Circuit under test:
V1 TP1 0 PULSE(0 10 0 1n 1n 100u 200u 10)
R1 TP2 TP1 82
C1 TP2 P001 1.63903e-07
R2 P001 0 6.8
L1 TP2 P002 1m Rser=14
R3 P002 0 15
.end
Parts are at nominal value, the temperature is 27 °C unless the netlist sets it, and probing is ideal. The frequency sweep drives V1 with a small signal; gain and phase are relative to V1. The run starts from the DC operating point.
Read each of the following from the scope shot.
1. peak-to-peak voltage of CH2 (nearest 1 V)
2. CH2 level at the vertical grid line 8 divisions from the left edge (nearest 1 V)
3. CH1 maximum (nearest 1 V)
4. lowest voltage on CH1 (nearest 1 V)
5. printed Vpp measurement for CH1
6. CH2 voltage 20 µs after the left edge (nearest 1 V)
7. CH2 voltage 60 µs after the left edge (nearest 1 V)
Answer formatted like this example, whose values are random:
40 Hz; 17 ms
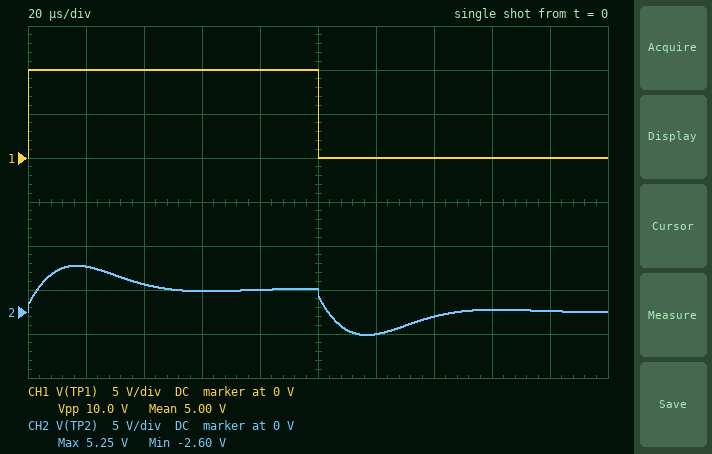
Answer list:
8 V; 0 V; 10 V; 0 V; 10.0 V; 5 V; 2 V
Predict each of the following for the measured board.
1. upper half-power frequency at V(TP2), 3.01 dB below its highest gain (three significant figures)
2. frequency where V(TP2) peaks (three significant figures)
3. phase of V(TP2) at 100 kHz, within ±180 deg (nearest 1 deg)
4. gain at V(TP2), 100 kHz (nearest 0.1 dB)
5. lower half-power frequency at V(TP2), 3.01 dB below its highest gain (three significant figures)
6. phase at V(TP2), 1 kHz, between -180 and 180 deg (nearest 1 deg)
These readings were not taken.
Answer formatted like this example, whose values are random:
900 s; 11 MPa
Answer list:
23.8 kHz; 13.4 kHz; -48 deg; -17.4 dB; 6.98 kHz; 8 deg
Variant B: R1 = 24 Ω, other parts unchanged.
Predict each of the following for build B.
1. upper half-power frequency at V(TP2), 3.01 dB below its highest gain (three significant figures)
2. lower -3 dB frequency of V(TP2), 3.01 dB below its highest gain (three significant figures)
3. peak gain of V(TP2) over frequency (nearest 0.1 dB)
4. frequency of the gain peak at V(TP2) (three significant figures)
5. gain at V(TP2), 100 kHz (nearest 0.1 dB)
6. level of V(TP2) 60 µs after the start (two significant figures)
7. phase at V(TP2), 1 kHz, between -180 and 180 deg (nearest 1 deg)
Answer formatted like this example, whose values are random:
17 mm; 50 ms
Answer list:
43.2 kHz; 3.29 kHz; -1.0 dB; 14.7 kHz; -8.6 dB; 5.7 V; 5 deg
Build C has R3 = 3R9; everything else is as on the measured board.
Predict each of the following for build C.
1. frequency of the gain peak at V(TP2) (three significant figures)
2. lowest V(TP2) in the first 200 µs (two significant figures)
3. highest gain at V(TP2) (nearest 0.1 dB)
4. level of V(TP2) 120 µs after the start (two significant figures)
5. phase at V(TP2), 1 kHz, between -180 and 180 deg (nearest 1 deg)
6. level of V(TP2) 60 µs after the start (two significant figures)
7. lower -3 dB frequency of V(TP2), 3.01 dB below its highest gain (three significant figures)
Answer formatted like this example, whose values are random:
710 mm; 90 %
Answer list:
13.0 kHz; -3.3 V; -2.4 dB; -3.2 V; 15 deg; 1.4 V; 7.41 kHz
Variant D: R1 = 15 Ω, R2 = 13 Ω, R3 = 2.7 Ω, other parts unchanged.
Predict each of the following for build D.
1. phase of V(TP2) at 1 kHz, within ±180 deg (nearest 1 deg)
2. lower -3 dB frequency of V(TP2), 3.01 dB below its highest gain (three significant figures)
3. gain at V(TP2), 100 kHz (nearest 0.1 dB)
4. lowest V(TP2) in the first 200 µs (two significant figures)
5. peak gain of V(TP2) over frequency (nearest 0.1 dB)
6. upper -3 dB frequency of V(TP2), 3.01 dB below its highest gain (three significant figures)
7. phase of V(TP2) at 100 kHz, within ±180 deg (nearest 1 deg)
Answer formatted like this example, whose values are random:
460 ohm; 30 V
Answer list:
9 deg; 2.62 kHz; -5.2 dB; -3.2 V; -0.6 dB; 56.7 kHz; -17 deg
